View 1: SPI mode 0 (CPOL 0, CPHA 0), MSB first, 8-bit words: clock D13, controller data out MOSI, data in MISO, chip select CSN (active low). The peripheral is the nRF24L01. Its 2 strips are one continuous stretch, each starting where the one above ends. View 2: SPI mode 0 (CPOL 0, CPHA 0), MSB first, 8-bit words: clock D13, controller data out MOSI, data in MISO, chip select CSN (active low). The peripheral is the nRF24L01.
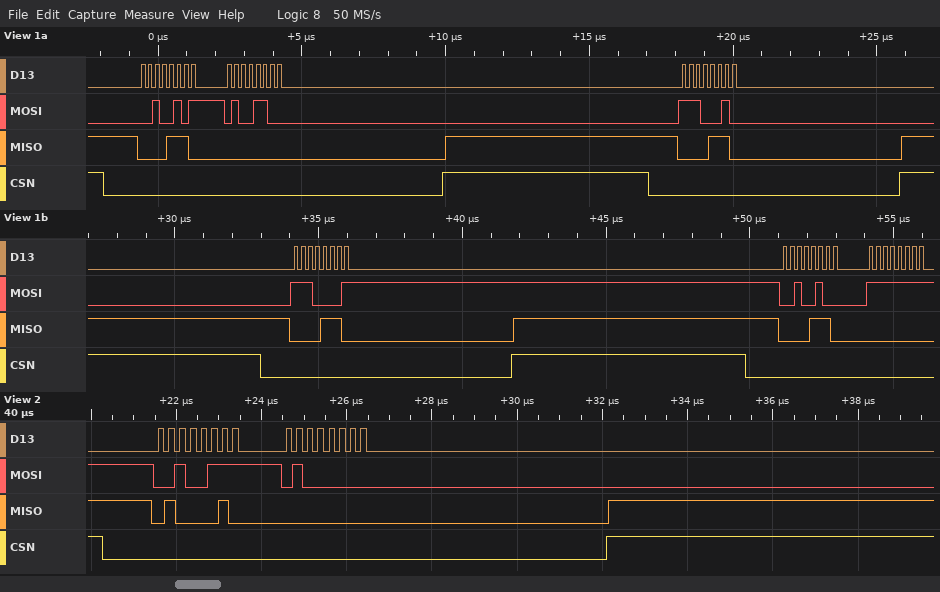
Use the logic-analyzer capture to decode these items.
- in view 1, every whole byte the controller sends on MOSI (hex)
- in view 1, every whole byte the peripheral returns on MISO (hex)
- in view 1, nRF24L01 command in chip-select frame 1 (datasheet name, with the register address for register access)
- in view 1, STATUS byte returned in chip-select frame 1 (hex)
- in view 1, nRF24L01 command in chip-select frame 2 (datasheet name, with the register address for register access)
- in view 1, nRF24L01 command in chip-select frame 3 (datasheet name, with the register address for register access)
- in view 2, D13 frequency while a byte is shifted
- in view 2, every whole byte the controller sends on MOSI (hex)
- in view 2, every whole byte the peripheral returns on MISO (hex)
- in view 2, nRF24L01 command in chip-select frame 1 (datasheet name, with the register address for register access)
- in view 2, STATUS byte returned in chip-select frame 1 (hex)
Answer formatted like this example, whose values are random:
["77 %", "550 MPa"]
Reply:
["0x25 0x4C 0xE2 0xE1 0x24 0xFF", "0x0E 0x00 0x0E 0x0E 0x0E 0x00", "W_REGISTER 0x05", "0x0E", "FLUSH_RX", "FLUSH_TX", "4 MHz", "27 40", "42 00", "W_REGISTER 0x07", "0x42"]
